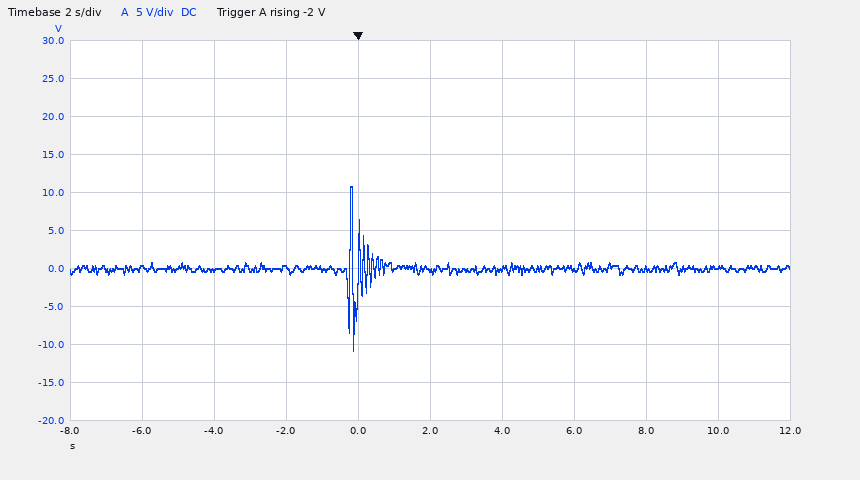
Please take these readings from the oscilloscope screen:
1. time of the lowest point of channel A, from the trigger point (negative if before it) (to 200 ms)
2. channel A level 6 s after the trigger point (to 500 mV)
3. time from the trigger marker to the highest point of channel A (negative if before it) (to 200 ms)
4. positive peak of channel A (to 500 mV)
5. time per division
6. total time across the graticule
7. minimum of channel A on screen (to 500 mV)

-200 ms
0.0 V
-200 ms
11.0 V
2 s
20 s
-11.0 V
